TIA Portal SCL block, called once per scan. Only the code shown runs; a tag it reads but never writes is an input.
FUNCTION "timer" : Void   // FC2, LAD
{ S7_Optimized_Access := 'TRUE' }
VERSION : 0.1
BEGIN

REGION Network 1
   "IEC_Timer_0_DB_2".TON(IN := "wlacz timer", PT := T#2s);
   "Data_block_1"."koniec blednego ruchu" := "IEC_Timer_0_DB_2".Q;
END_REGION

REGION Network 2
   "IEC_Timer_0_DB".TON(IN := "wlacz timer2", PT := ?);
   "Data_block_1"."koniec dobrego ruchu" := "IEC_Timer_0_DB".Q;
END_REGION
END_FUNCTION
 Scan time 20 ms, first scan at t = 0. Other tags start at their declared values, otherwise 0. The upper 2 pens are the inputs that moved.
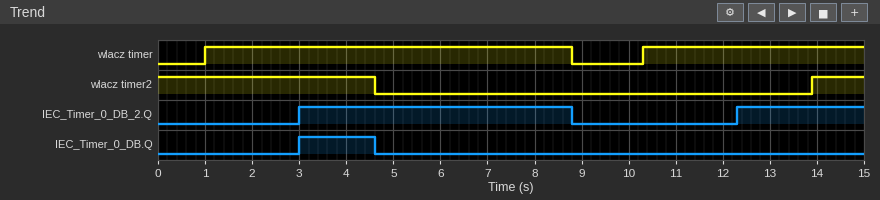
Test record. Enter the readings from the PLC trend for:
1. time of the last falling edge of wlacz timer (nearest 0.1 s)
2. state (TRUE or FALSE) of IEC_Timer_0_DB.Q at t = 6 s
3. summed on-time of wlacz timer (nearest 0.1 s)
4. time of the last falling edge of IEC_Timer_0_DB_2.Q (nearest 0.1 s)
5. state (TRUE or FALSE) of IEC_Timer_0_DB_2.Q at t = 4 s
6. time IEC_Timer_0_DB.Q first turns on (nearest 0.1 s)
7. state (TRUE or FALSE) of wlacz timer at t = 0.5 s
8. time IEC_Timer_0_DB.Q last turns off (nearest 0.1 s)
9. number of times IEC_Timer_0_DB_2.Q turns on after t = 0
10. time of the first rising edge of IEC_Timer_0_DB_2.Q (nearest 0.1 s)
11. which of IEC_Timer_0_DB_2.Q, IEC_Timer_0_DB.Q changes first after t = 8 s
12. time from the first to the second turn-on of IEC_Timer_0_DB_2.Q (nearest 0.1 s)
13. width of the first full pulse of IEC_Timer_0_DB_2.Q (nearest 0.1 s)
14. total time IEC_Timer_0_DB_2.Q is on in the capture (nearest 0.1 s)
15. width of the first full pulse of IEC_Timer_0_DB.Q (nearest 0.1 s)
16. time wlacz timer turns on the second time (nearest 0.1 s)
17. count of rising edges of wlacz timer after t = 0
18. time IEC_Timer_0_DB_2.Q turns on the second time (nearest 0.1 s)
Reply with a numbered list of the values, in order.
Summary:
1. 8.8 s
2. FALSE
3. 12.5 s
4. 8.8 s
5. TRUE
6. 3.0 s
7. FALSE
8. 4.6 s
9. 2
10. 3.0 s
11. IEC_Timer_0_DB_2.Q
12. 9.3 s
13. 5.8 s
14. 8.5 s
15. 1.6 s
16. 10.3 s
17. 2
18. 12.3 s
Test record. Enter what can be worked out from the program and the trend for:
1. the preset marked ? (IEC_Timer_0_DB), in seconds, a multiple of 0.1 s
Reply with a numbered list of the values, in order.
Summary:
1. 3.0 s
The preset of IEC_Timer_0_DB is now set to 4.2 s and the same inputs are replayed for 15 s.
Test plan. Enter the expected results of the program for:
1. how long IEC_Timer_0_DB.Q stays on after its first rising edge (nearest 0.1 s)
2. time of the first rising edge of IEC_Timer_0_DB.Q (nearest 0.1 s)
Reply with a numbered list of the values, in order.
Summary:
1. 0.4 s
2. 4.2 s
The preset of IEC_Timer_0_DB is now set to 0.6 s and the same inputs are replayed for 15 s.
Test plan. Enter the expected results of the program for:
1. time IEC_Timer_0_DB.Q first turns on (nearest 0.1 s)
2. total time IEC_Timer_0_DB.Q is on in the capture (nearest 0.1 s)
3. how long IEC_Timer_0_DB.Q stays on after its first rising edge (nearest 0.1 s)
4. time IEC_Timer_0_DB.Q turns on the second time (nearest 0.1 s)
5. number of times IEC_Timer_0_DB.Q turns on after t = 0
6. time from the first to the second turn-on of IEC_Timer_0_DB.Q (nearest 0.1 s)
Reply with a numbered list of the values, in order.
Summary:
1. 0.6 s
2. 4.5 s
3. 4.0 s
4. 14.5 s
5. 2
6. 13.9 s
